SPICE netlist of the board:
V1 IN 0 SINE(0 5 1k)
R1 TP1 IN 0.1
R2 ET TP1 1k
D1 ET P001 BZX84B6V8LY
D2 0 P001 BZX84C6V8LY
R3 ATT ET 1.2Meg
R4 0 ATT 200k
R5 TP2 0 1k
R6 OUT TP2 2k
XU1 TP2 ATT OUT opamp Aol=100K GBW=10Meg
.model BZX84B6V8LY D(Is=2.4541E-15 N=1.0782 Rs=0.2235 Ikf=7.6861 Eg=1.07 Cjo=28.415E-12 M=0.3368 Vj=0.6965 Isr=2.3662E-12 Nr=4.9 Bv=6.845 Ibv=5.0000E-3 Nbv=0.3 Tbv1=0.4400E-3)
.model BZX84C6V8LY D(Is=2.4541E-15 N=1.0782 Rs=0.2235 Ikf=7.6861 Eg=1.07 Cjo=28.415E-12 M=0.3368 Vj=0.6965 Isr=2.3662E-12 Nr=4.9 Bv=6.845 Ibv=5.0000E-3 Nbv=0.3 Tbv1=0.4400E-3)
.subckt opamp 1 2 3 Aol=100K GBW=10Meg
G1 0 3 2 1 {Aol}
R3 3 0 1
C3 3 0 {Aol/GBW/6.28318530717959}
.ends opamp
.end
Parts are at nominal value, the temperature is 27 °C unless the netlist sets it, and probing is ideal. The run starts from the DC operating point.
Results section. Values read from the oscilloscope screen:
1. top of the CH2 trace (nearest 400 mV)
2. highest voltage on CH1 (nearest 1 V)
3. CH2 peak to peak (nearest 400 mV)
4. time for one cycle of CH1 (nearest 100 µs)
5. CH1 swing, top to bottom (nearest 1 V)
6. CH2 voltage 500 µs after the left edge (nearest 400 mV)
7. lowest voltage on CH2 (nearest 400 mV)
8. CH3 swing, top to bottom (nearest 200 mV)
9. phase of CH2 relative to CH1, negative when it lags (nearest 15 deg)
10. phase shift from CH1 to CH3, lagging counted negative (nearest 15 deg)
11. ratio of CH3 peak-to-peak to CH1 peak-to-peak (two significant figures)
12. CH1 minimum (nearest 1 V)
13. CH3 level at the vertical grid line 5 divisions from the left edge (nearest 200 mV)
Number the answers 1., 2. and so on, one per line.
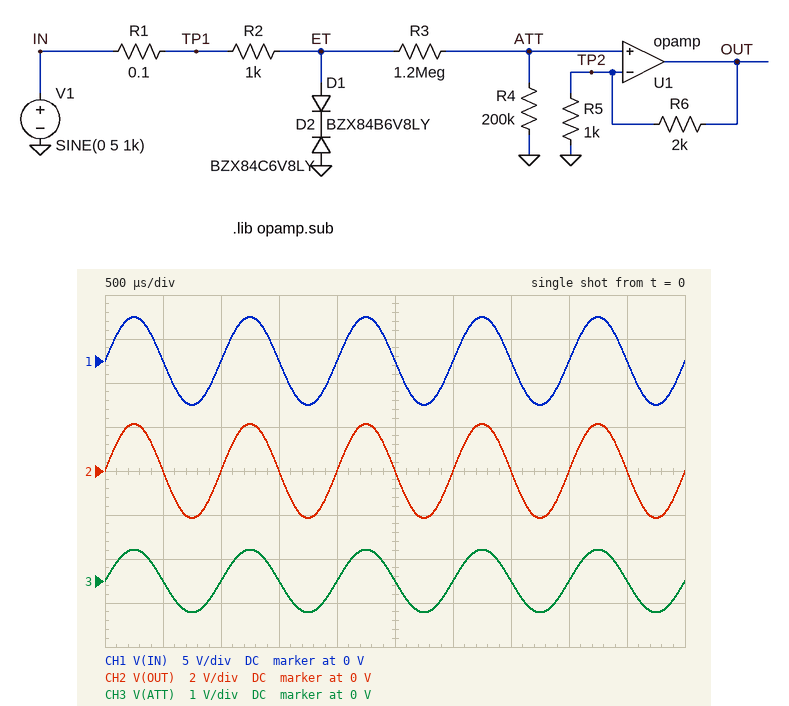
1. 2.0 V
2. 5 V
3. 4.4 V
4. 1.0 ms
5. 10 V
6. 0 V
7. -2.0 V
8. 1.4 V
9. 0 deg
10. 0 deg
11. 0.14
12. -5 V
13. 0 V
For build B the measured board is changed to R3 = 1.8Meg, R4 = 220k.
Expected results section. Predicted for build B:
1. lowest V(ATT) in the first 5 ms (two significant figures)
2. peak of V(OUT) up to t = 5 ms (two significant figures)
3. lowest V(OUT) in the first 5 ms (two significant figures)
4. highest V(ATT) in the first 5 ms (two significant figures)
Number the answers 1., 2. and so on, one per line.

1. -540 mV
2. 1.6 V
3. -1.6 V
4. 540 mV
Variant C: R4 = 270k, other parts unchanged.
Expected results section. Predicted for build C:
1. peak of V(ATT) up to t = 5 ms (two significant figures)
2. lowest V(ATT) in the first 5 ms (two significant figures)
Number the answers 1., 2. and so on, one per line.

1. 920 mV
2. -920 mV
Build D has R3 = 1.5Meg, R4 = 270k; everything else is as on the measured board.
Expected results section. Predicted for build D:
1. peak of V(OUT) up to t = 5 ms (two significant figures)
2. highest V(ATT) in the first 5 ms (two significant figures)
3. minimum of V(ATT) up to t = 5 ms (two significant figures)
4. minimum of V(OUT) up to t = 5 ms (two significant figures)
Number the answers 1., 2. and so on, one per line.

1. 2.3 V
2. 760 mV
3. -760 mV
4. -2.3 V
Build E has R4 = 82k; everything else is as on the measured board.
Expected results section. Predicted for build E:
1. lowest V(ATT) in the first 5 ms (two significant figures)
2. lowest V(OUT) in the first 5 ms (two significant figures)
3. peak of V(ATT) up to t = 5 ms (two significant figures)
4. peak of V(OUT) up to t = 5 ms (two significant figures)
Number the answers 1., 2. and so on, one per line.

1. -320 mV
2. -960 mV
3. 320 mV
4. 960 mV
